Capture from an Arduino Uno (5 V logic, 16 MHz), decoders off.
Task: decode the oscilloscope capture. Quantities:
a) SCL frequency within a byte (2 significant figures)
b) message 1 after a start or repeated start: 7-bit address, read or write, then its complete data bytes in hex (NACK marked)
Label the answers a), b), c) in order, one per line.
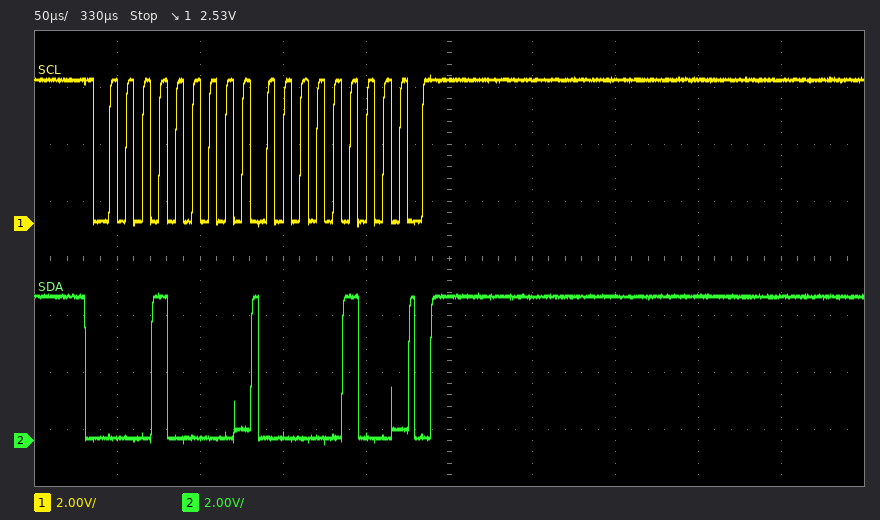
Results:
a) 100 kHz
b) 0x08 write: 04
